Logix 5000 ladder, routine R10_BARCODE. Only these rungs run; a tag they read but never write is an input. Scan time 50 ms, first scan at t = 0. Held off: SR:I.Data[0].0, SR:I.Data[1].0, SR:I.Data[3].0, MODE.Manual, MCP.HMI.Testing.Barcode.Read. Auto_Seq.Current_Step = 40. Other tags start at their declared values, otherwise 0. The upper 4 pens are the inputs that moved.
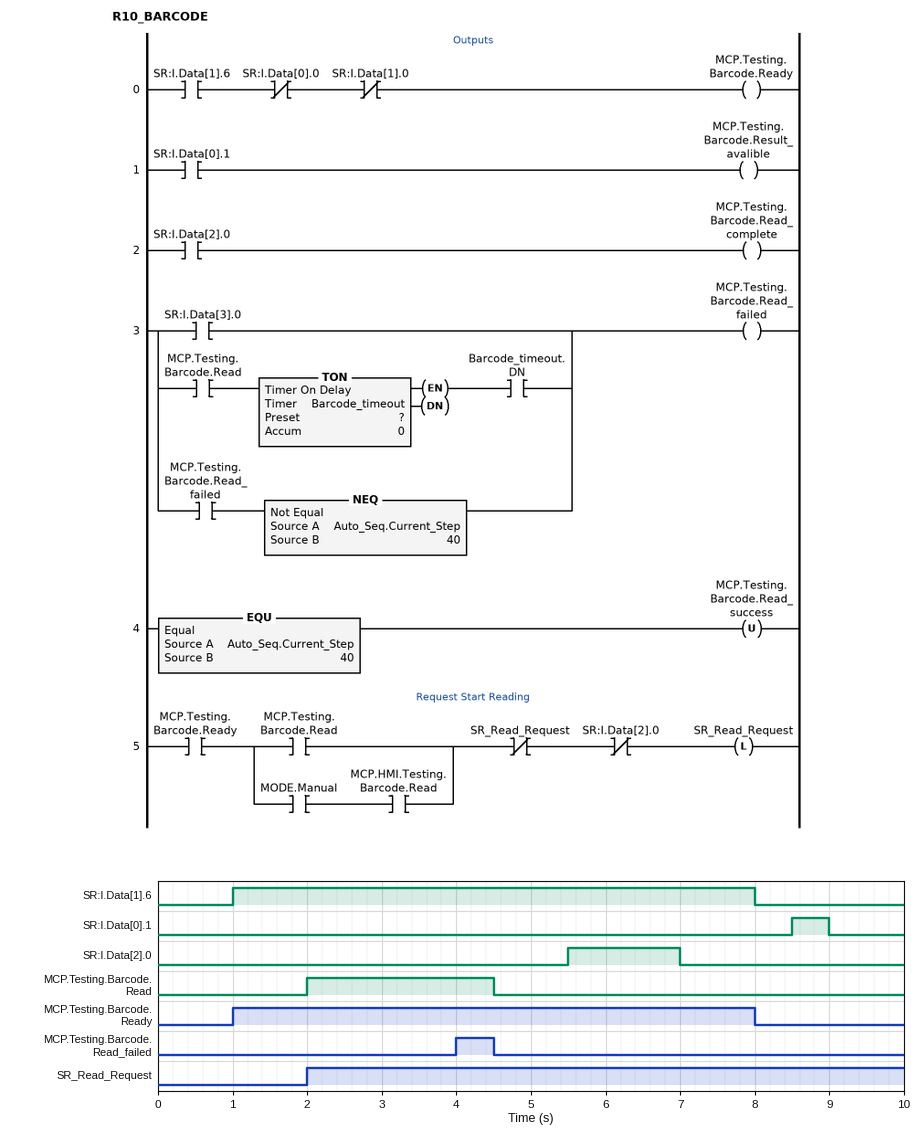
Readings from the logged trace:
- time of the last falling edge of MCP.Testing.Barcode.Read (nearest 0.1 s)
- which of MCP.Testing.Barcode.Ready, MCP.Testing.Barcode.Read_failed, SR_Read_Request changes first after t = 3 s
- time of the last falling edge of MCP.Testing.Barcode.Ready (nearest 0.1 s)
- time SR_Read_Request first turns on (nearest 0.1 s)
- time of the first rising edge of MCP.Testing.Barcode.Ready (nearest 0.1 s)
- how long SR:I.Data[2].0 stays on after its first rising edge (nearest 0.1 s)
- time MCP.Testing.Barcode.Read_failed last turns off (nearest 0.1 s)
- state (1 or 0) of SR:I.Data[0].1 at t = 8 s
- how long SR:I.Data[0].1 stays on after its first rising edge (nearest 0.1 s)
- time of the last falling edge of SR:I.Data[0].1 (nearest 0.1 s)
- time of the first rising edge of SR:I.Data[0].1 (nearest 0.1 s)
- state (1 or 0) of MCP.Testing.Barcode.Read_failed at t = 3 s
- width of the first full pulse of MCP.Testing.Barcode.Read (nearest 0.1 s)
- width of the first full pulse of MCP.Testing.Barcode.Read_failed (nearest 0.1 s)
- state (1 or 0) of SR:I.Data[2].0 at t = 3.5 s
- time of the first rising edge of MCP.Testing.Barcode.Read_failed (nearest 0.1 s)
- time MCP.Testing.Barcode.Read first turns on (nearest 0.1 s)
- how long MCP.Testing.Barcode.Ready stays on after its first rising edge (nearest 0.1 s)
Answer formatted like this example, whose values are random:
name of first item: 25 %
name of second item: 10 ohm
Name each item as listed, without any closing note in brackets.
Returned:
time of the last falling edge of MCP.Testing.Barcode.Read: 4.5 s
which of MCP.Testing.Barcode.Ready, MCP.Testing.Barcode.Read_failed, SR_Read_Request changes first after t = 3 s: MCP.Testing.Barcode.Read_failed
time of the last falling edge of MCP.Testing.Barcode.Ready: 8.0 s
time SR_Read_Request first turns on: 2.0 s
time of the first rising edge of MCP.Testing.Barcode.Ready: 1.0 s
how long SR:I.Data[2].0 stays on after its first rising edge: 1.5 s
time MCP.Testing.Barcode.Read_failed last turns off: 4.5 s
state (1 or 0) of SR:I.Data[0].1 at t = 8 s: 0
how long SR:I.Data[0].1 stays on after its first rising edge: 0.5 s
time of the last falling edge of SR:I.Data[0].1: 9.0 s
time of the first rising edge of SR:I.Data[0].1: 8.5 s
state (1 or 0) of MCP.Testing.Barcode.Read_failed at t = 3 s: 0
width of the first full pulse of MCP.Testing.Barcode.Read: 2.5 s
width of the first full pulse of MCP.Testing.Barcode.Read_failed: 0.5 s
state (1 or 0) of SR:I.Data[2].0 at t = 3.5 s: 0
time of the first rising edge of MCP.Testing.Barcode.Read_failed: 4.0 s
time MCP.Testing.Barcode.Read first turns on: 2.0 s
how long MCP.Testing.Barcode.Ready stays on after its first rising edge: 7.0 s
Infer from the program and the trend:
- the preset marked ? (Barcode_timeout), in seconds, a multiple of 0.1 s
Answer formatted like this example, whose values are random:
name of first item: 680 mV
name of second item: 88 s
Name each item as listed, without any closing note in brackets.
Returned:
the preset marked ? (Barcode_timeout), in seconds, a multiple of 0.1 s: 2.0 s
